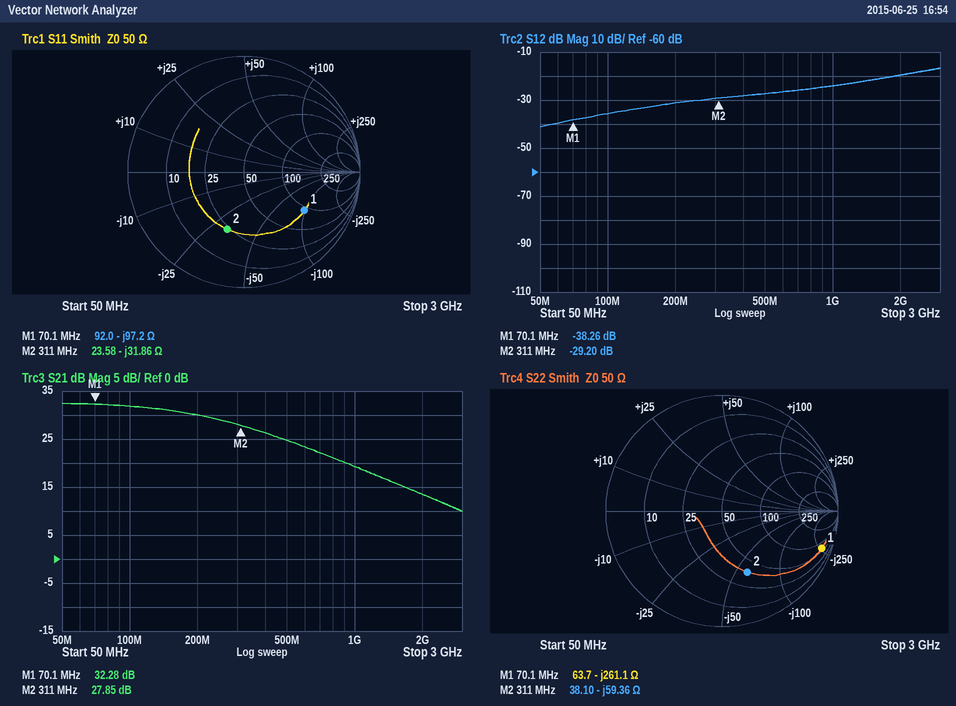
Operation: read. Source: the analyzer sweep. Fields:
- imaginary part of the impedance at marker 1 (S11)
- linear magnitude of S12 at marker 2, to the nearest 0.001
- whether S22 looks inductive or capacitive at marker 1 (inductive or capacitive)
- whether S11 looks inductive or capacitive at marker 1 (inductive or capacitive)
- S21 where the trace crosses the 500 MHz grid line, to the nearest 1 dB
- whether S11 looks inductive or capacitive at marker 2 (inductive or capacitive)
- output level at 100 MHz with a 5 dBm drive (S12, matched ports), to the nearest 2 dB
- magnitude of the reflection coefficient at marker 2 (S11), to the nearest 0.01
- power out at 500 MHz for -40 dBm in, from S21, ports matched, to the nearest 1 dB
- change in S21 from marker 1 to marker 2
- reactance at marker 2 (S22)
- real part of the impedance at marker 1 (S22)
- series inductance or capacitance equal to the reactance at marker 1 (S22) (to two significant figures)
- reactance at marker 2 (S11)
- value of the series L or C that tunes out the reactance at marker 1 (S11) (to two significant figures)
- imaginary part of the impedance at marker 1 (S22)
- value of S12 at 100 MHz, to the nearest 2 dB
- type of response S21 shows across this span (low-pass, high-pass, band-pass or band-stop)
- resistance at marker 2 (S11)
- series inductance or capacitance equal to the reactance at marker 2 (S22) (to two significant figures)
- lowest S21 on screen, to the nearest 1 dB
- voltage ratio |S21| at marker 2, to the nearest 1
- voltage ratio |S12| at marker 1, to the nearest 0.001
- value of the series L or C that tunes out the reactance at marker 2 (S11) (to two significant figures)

-97.2 Ω
0.035
capacitive
capacitive
25 dB
capacitive
-30 dBm
0.52
-15 dBm
-4.43 dB
-59.36 Ω
63.7 Ω
8.7 pF
-31.86 Ω
220 nH
-261.1 Ω
-36 dB
low-pass
23.58 Ω
8.6 pF
10 dB
25
0.012
16 nH
